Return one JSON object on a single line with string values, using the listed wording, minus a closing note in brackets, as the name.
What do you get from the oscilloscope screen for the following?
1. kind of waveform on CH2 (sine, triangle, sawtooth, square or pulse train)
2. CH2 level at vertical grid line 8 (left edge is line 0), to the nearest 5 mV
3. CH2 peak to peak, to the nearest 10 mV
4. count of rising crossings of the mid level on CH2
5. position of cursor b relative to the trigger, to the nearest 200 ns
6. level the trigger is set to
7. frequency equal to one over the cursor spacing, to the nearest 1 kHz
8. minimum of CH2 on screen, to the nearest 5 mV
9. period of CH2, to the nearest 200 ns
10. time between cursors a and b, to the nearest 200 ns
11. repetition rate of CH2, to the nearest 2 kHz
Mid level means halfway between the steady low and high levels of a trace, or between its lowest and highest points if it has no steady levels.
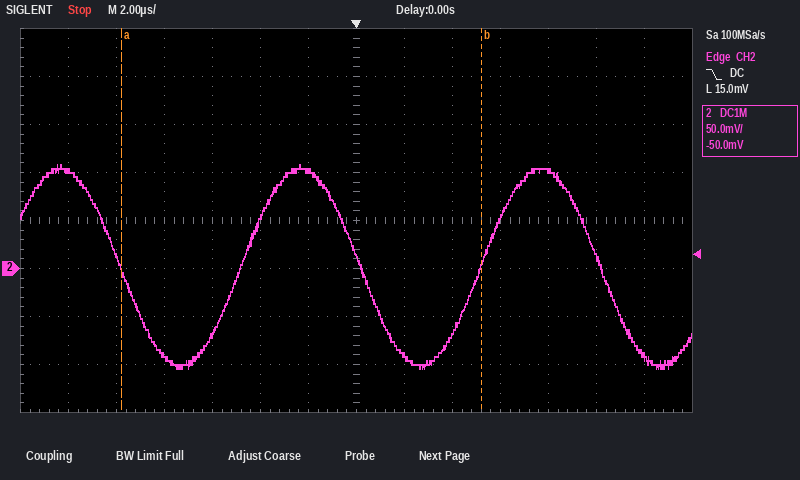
{"kind of waveform on CH2": "sine", "CH2 level at vertical grid line 8 (left edge is line 0), to the nearest 5 mV": "-90 mV", "CH2 peak to peak, to the nearest 10 mV": "210 mV", "count of rising crossings of the mid level on CH2": "2", "position of cursor b relative to the trigger, to the nearest 200 ns": "+5.2 µs", "level the trigger is set to": "15.0 mV", "frequency equal to one over the cursor spacing, to the nearest 1 kHz": "67 kHz", "minimum of CH2 on screen, to the nearest 5 mV": "-105 mV", "period of CH2, to the nearest 200 ns": "10.0 µs", "time between cursors a and b, to the nearest 200 ns": "15.0 µs", "repetition rate of CH2, to the nearest 2 kHz": "100 kHz"}
